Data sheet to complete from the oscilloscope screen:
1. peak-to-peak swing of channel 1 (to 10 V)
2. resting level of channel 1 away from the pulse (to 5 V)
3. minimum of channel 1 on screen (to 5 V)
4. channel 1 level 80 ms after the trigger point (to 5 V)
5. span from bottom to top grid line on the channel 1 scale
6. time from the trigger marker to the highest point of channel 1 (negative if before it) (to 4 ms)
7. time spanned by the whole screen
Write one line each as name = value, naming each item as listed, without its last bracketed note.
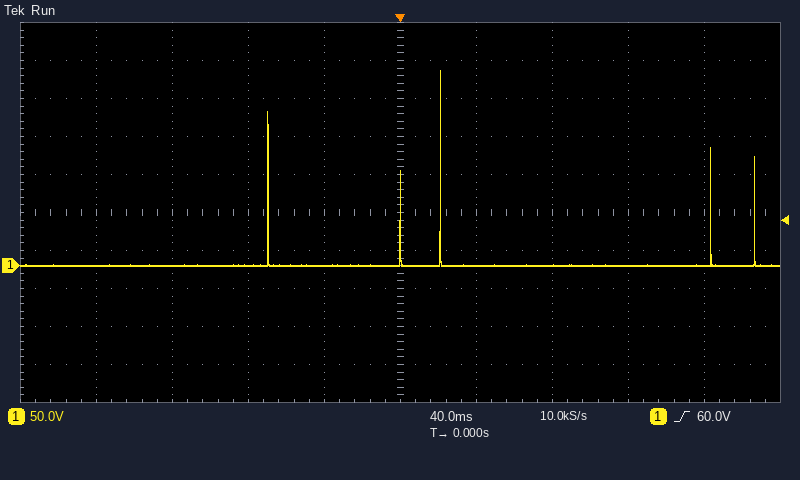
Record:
peak-to-peak swing of channel 1 = 260 V
resting level of channel 1 away from the pulse = 0 V
minimum of channel 1 on screen = 0 V
channel 1 level 80 ms after the trigger point = 0 V
span from bottom to top grid line on the channel 1 scale = 500 V
time from the trigger marker to the highest point of channel 1 (negative if before it) = +20 ms
time spanned by the whole screen = 400 ms
